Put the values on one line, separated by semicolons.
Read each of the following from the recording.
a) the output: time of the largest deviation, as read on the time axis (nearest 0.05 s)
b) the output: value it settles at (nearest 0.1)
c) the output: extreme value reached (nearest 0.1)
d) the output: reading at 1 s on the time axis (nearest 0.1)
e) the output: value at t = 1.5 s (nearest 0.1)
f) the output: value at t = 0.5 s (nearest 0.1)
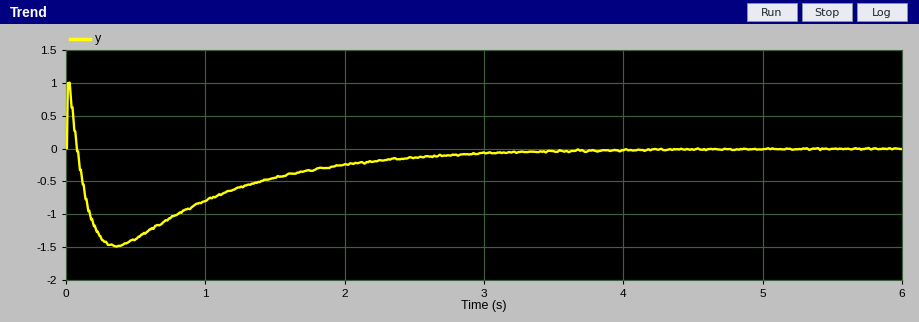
0.35 s; 0.0; -1.5; -0.8; -0.4; -1.4
